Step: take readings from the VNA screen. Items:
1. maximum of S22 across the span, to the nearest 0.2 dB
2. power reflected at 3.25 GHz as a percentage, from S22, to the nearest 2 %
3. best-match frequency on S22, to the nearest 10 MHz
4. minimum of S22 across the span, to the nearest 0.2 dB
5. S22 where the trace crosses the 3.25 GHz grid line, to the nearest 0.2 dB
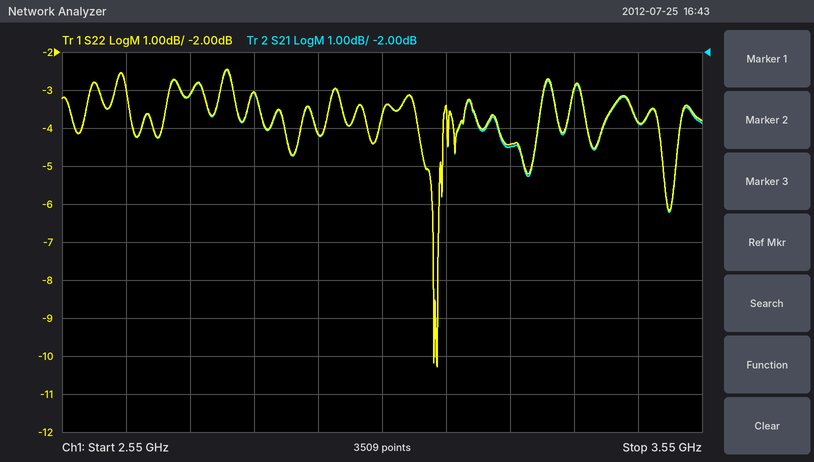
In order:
-2.4 dB
36 %
3.14 GHz
-10.2 dB
-4.4 dB
